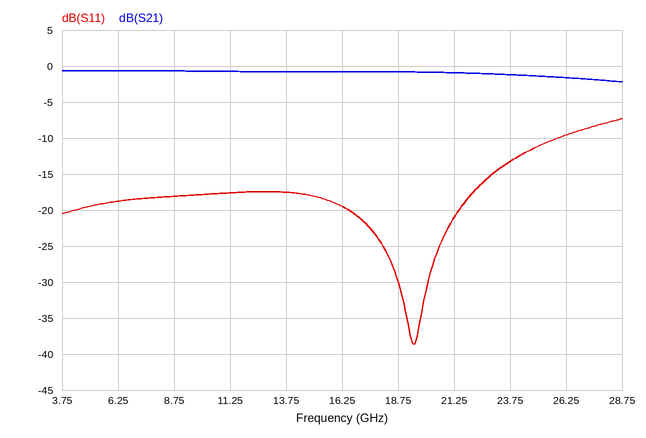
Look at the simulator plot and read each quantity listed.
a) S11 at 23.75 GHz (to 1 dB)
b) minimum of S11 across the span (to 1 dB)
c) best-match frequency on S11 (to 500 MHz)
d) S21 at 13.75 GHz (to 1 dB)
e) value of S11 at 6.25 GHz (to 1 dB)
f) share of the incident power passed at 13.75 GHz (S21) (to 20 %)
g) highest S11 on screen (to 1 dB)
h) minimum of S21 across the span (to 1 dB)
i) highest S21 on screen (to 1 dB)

-13 dB
-39 dB
19.5 GHz
-1 dB
-19 dB
80 %
-7 dB
-2 dB
-1 dB
